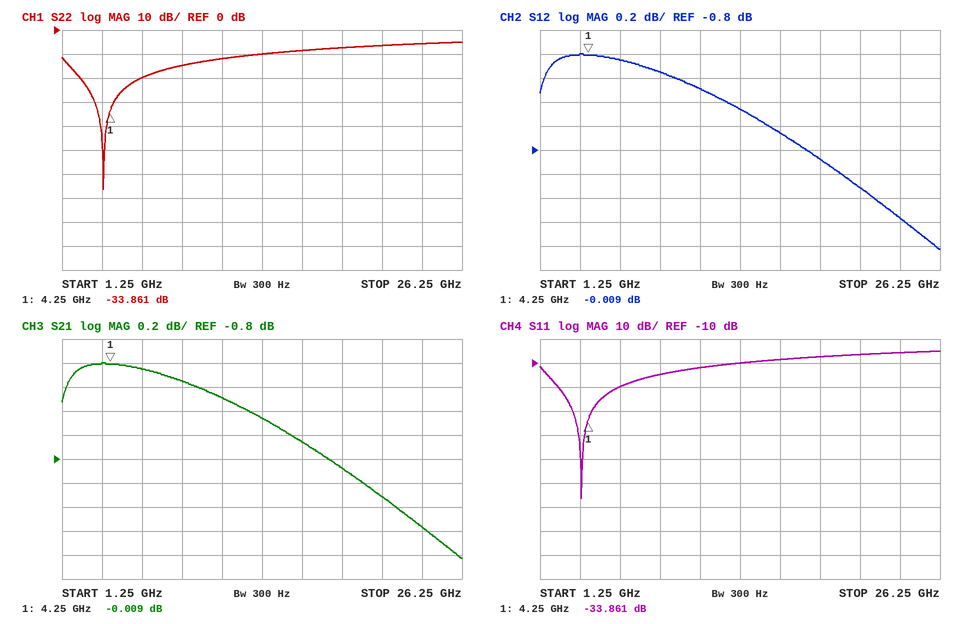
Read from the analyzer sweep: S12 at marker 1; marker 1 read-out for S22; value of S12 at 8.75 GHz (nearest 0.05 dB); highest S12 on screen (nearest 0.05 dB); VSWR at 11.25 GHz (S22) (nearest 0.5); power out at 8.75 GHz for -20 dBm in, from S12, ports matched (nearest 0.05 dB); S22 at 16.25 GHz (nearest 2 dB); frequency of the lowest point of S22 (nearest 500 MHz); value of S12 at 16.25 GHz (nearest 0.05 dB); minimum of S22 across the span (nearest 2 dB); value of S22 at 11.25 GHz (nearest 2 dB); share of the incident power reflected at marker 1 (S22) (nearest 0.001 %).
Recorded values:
-0.009 dB
-33.861 dB
-0.15 dB
0.00 dB
1.5
-20.15 dBm
-8 dB
4.0 GHz
-0.65 dB
-66 dB
-12 dB
0.041 %
